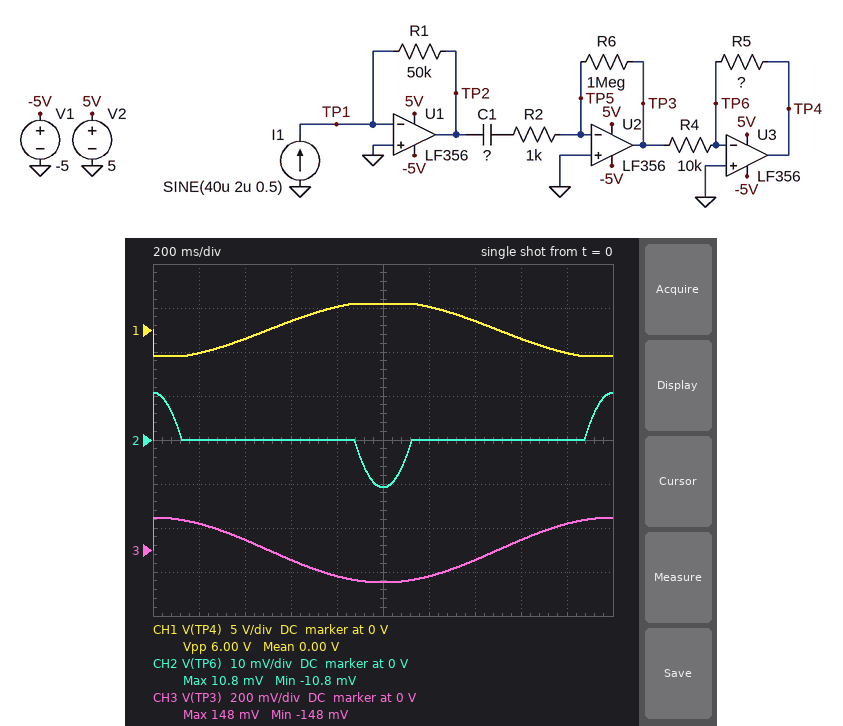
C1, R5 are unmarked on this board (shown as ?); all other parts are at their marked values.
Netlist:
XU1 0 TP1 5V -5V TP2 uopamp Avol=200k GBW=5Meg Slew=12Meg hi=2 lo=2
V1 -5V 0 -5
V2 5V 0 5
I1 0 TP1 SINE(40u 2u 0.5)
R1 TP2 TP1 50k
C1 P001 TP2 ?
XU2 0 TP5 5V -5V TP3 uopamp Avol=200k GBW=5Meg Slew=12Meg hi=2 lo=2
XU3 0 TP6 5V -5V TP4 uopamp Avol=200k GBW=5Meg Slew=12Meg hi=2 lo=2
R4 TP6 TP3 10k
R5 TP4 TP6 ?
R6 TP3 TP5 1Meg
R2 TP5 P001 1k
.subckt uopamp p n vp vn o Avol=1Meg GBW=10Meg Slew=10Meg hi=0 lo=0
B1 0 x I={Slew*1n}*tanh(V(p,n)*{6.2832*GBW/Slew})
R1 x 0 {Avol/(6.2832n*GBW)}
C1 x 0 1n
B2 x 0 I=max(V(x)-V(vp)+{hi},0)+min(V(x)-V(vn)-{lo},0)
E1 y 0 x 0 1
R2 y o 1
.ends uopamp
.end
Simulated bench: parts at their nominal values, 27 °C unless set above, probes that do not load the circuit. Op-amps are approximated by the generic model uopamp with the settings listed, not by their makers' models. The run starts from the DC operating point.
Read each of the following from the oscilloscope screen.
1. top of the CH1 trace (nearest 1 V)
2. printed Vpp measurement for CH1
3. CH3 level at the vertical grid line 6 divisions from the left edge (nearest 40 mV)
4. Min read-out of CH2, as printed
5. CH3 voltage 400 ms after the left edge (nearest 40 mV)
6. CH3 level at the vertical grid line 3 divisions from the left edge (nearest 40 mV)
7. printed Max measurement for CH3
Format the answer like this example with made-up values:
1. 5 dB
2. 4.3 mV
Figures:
1. 3 V
2. 6.00 V
3. -120 mV
4. -10.8 mV
5. 40 mV
6. -40 mV
7. 148 mV
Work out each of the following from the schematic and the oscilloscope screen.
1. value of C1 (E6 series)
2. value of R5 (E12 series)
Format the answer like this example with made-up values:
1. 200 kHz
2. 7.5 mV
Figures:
1. 470 nF
2. 220 kΩ
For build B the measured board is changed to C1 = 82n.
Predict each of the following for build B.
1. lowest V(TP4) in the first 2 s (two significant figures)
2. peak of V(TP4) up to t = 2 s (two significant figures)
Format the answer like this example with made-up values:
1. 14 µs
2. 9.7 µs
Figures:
1. -580 mV
2. 570 mV
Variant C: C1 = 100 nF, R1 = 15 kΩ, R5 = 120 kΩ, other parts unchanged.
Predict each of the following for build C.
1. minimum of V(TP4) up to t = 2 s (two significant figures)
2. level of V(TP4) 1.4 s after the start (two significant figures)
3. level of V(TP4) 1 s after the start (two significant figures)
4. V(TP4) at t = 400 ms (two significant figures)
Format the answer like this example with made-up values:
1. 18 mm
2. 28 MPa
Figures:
1. -110 mV
2. 35 mV
3. 110 mV
4. -35 mV
